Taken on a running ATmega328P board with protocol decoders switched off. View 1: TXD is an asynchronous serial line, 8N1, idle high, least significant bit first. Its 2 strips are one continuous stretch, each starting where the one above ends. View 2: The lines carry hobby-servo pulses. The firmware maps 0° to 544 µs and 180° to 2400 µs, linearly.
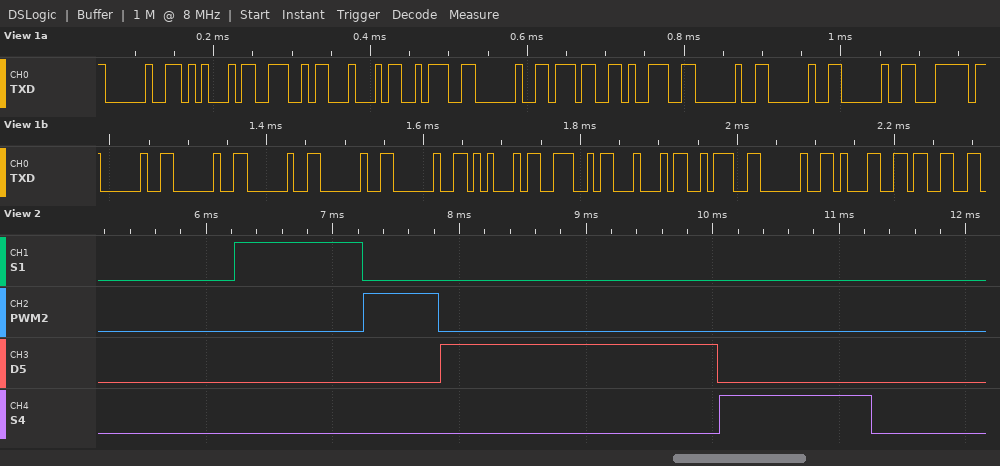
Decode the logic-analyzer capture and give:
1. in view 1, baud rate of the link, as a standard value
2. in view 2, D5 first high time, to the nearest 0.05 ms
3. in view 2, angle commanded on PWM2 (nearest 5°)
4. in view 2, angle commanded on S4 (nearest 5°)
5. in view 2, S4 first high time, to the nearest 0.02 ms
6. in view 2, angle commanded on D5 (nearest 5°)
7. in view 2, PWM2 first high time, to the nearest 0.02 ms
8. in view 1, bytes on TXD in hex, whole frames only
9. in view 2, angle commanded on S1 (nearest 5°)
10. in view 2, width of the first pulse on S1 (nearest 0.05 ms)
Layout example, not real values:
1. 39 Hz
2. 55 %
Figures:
1. 115200 baud
2. 2.20 ms
3. 5°
4. 65°
5. 1.20 ms
6. 160°
7. 0.60 ms
8. 20 45 4E 44 3A 20 37 39 20 20 20 7C 20 20 20 20 20 45 4E 44 3A 20 31 33
9. 45°
10. 1.00 ms
